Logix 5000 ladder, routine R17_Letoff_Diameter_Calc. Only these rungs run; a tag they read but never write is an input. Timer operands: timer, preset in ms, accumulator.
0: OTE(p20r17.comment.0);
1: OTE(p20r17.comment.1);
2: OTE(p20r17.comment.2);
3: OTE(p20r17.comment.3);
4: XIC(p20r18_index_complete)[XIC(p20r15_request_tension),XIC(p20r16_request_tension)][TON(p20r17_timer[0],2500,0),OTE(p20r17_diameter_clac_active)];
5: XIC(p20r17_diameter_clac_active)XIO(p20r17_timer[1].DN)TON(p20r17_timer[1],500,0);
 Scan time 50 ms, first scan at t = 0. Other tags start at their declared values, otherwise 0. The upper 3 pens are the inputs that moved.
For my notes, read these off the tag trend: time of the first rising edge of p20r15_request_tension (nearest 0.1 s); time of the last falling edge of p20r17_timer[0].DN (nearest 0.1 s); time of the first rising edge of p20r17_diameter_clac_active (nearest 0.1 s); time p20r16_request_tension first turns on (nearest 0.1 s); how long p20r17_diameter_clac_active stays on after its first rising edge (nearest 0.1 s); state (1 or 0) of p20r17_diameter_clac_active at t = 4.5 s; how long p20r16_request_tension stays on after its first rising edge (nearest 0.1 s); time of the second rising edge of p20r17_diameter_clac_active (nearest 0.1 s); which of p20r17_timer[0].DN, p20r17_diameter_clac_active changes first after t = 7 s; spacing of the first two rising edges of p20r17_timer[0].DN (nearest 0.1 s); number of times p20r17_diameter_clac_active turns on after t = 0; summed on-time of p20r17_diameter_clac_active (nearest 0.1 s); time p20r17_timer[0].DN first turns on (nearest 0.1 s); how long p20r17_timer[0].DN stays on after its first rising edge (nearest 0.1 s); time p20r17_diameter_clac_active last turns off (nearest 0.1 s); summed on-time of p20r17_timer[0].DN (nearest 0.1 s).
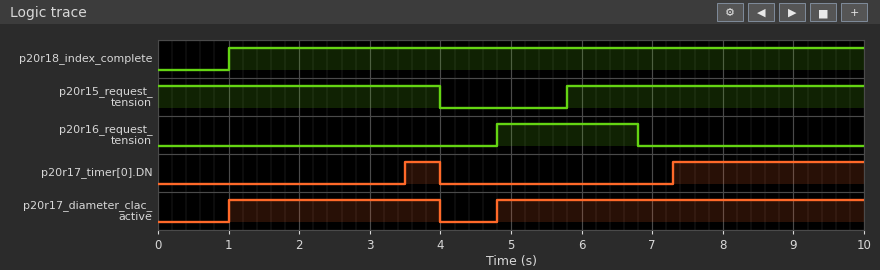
5.8 s
4.0 s
1.0 s
4.8 s
3.0 s
0
2.0 s
4.8 s
p20r17_timer[0].DN
3.8 s
2
8.2 s
3.5 s
0.5 s
4.0 s
3.2 s
